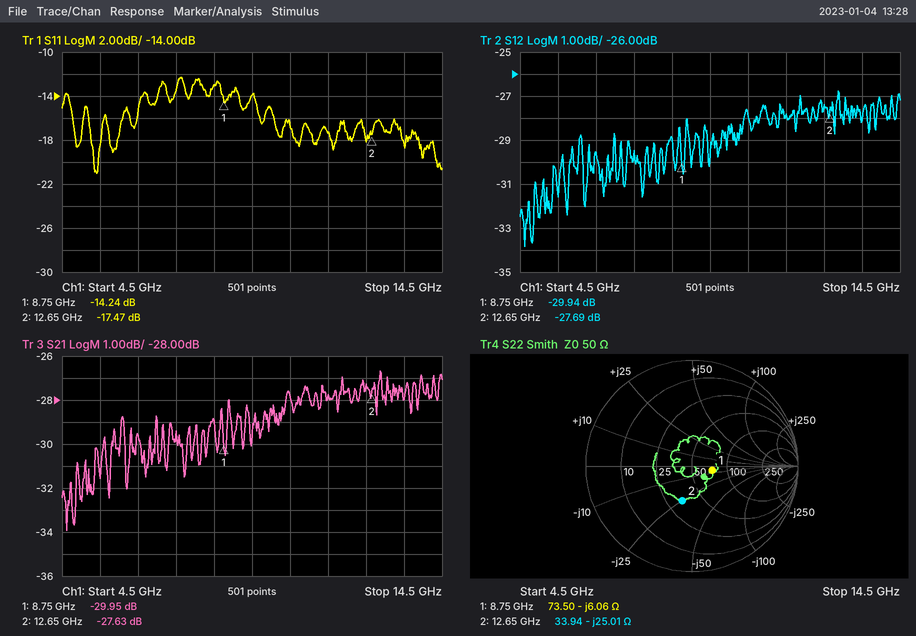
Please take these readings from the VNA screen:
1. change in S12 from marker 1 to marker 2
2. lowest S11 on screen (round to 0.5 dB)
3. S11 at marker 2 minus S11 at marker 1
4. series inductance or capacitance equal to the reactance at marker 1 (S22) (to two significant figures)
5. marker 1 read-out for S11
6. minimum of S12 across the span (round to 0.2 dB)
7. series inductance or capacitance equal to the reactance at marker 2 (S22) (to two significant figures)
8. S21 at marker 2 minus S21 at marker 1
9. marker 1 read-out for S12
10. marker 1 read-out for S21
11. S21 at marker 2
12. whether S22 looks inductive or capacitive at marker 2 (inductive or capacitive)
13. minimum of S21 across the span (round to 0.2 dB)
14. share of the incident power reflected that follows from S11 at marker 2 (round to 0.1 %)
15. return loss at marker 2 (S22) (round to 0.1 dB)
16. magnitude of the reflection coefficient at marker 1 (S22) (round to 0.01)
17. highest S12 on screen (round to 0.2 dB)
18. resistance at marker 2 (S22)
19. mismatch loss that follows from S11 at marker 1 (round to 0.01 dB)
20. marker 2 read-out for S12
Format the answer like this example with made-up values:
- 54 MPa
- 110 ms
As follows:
- 2.25 dB
- -21.0 dB
- -3.23 dB
- 3.0 pF
- -14.24 dB
- -33.8 dB
- 500 fF
- 2.32 dB
- -29.94 dB
- -29.95 dB
- -27.63 dB
- capacitive
- -34.0 dB
- 1.8 %
- 9.4 dB
- 0.20
- -26.8 dB
- 33.94 Ω
- 0.17 dB
- -27.69 dB
